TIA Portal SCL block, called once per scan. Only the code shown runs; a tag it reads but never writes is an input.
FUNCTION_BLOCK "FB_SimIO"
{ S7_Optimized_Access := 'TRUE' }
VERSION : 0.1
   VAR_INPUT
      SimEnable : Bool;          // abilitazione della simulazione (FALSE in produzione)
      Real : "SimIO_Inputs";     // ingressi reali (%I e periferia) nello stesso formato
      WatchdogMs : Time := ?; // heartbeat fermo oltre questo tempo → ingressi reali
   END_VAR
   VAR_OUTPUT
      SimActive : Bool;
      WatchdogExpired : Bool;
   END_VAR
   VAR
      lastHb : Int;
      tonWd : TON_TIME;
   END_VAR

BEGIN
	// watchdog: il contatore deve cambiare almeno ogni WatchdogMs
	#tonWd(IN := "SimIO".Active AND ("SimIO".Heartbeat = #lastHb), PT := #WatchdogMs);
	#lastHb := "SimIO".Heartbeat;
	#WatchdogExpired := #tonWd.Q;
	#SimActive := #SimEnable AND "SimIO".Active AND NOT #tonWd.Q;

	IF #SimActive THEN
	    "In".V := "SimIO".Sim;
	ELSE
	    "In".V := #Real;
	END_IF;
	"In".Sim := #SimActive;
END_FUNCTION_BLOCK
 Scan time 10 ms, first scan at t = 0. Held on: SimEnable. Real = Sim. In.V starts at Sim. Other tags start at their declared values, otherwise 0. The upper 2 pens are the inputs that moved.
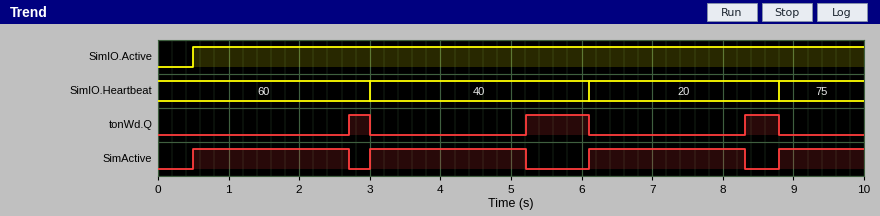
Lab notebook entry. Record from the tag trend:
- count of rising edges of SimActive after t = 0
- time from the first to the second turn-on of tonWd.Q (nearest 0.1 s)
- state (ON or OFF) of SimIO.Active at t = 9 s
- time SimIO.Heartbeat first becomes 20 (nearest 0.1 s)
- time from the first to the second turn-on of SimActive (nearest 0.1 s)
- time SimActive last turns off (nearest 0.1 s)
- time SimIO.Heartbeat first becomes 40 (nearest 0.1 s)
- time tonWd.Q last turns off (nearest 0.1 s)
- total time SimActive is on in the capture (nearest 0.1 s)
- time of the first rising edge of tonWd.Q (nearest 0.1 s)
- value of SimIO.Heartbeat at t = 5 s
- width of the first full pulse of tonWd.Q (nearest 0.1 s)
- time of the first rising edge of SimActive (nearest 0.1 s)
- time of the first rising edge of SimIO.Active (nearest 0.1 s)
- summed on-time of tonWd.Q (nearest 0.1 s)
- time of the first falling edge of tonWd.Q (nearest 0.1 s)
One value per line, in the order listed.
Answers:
4
2.5 s
ON
6.1 s
2.5 s
8.3 s
3.0 s
8.8 s
7.8 s
2.7 s
40
0.3 s
0.5 s
0.5 s
1.7 s
3.0 s
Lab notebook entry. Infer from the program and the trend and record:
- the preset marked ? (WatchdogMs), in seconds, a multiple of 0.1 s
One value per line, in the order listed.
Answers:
2.2 s
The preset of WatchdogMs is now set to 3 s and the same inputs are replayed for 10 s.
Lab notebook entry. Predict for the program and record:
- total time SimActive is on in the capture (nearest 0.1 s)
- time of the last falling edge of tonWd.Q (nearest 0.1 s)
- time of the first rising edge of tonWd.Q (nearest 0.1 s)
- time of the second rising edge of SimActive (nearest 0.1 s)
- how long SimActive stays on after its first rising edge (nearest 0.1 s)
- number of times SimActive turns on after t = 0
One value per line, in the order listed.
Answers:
9.4 s
6.1 s
6.0 s
6.1 s
5.5 s
2
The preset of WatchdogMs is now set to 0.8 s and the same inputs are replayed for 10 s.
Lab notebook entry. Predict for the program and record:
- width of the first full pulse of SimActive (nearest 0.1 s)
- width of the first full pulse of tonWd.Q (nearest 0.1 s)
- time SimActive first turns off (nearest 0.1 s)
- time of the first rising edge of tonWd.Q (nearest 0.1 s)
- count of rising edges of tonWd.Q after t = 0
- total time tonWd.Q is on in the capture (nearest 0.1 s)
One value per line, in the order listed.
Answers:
0.8 s
1.7 s
1.3 s
1.3 s
4
6.3 s
